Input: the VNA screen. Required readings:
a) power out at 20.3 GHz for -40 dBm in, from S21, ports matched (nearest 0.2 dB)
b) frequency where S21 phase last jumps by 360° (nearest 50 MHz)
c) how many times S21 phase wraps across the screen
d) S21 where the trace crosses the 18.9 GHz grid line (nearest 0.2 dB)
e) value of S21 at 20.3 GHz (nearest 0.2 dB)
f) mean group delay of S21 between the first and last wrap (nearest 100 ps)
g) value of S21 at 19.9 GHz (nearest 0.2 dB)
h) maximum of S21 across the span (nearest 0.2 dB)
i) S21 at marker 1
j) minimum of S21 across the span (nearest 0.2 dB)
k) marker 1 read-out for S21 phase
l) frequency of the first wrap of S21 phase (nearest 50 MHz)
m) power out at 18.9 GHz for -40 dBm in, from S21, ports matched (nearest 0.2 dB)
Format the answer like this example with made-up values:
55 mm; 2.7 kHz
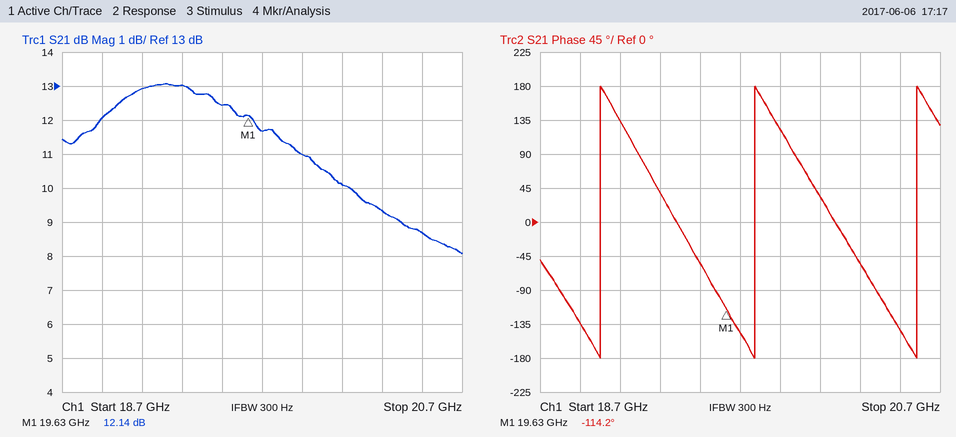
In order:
-30.6 dBm; 20.60 GHz; 3; 12.0 dB; 9.4 dB; 1.3 ns; 11.0 dB; 13.0 dB; 12.14 dB; 8.0 dB; -114.2°; 19.00 GHz; -28.0 dBm
